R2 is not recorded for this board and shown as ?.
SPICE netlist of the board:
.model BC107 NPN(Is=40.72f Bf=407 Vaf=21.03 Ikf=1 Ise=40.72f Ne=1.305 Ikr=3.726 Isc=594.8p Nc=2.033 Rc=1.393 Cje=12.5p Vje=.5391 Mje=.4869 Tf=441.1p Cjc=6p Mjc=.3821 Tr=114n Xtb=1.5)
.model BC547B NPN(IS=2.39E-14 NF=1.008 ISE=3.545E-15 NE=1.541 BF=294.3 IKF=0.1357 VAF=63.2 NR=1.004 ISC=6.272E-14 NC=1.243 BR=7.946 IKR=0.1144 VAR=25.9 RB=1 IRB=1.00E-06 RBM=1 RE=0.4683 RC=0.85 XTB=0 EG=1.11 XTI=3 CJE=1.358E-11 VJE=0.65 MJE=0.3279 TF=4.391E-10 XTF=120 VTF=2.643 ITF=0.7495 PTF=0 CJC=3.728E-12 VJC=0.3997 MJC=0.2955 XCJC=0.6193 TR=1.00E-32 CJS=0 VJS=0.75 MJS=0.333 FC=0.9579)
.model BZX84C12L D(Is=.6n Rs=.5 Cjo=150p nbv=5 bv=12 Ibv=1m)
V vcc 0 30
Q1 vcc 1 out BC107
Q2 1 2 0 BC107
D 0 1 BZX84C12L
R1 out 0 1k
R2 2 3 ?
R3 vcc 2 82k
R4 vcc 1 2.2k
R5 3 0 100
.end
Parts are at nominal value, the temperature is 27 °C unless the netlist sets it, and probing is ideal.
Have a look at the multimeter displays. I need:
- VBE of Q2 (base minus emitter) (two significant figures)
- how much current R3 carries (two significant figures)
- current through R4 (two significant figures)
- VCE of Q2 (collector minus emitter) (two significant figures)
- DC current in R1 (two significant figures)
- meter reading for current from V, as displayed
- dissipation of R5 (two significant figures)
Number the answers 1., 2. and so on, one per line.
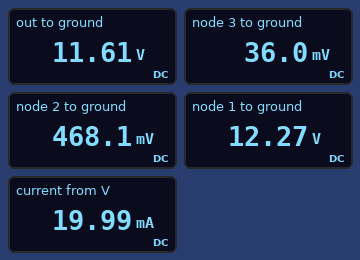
1. 470 mV
2. 360 µA
3. 8.1 mA
4. 12 V
5. 12 mA
6. 19.99 mA
7. 13 µW
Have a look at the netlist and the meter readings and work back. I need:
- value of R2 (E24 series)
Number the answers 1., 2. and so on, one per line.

1. 1.2 kΩ
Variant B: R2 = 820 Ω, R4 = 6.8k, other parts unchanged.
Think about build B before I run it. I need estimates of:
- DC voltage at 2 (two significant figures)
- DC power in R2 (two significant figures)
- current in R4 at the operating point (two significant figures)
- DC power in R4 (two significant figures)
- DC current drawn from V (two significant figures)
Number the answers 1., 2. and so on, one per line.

1. 330 mV
2. 110 µW
3. 2.6 mA
4. 47 mW
5. 14 mA
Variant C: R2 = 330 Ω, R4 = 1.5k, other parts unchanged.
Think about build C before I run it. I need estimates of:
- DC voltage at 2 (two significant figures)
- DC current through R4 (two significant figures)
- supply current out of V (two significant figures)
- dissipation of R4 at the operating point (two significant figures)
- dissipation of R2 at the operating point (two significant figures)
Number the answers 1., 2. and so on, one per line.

1. 160 mV
2. 12 mA
3. 24 mA
4. 210 mW
5. 44 µW
